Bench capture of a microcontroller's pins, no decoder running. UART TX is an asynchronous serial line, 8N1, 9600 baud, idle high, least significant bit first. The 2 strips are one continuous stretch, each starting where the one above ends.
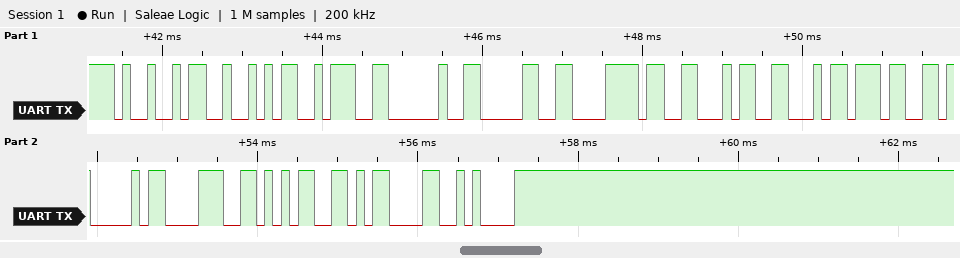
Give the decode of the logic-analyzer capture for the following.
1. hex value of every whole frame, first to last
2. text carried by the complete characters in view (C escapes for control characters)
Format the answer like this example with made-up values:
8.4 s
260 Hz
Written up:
0x49 0x52 0x3A 0x20 0x30 0x78 0x46 0x46 0x37 0x41 0x38 0x35 0x0D 0x0A
"IR: 0xFF7A85\r\n"
